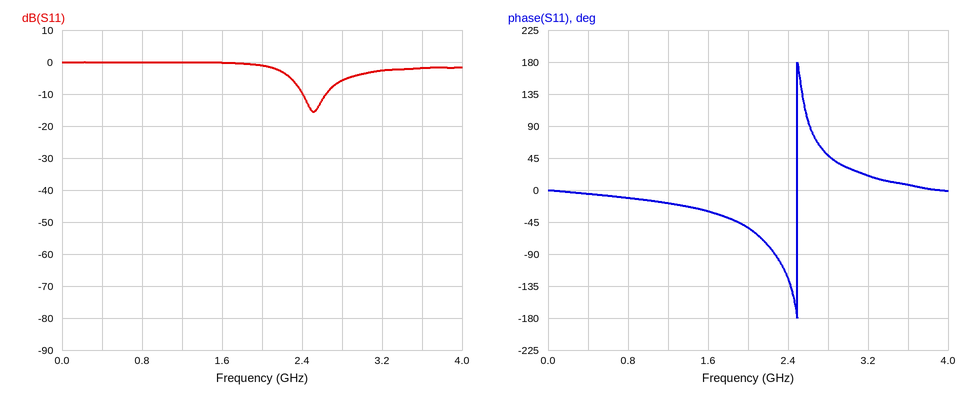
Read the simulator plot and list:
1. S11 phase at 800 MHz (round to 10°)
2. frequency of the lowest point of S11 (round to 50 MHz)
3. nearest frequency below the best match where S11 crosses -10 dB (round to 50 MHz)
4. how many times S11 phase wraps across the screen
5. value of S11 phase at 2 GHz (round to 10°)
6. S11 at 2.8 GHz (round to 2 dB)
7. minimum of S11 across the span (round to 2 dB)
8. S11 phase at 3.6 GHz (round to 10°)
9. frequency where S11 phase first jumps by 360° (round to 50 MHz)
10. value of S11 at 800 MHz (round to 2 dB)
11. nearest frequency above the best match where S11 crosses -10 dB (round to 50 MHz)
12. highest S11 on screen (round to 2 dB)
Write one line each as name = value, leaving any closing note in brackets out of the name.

S11 phase at 800 MHz = -10°
frequency of the lowest point of S11 = 2.50 GHz
nearest frequency below the best match where S11 crosses -10 dB = 2.40 GHz
how many times S11 phase wraps across the screen = 1
value of S11 phase at 2 GHz = -50°
S11 at 2.8 GHz = -6 dB
minimum of S11 across the span = -16 dB
S11 phase at 3.6 GHz = 10°
frequency where S11 phase first jumps by 360° = 2.50 GHz
value of S11 at 800 MHz = 0 dB
nearest frequency above the best match where S11 crosses -10 dB = 2.65 GHz
highest S11 on screen = 0 dB
